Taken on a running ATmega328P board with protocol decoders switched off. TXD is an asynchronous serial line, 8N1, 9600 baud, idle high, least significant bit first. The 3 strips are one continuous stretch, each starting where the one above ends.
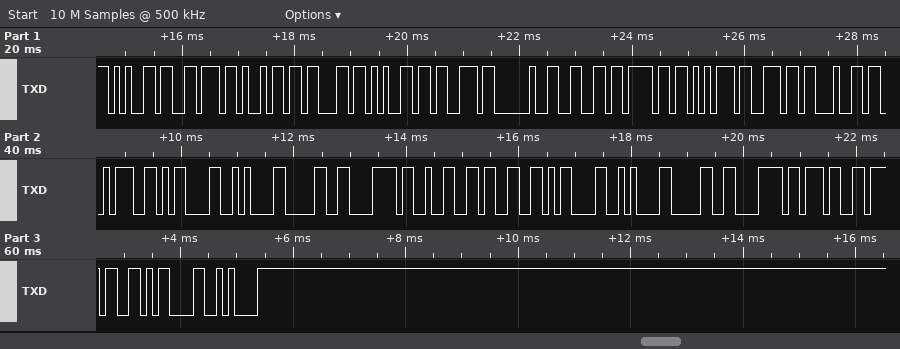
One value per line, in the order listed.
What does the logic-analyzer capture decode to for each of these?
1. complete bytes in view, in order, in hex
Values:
65 76 69 63 65 73 20 66 6F 75 6E 64 3A 0D 0A 30 78 32 33 0D 0A 30 78 37 37 0D 0A
